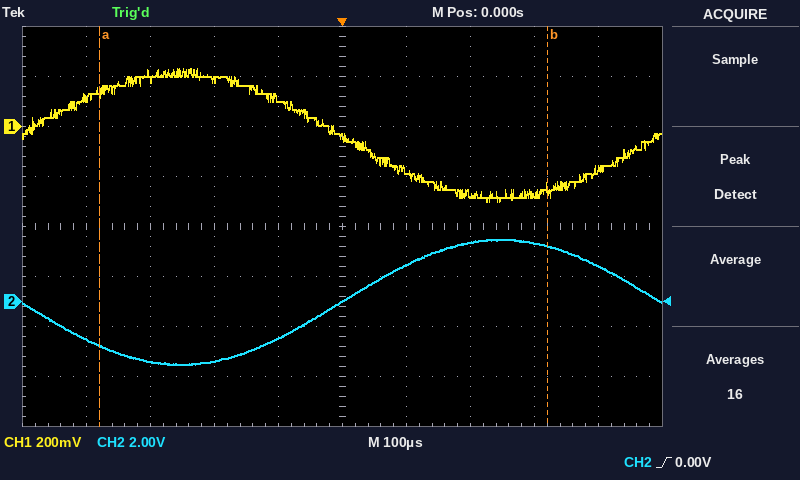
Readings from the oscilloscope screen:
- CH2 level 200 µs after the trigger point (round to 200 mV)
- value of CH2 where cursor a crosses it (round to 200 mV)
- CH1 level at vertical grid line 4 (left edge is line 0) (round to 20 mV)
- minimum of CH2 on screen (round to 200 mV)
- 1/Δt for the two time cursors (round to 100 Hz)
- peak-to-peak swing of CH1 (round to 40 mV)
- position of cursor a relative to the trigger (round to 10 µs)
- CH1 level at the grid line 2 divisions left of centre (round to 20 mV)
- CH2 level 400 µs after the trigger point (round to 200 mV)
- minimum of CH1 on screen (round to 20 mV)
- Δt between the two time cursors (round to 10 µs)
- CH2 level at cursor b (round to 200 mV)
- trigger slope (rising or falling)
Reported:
2.4 V
-1.8 V
120 mV
-2.6 V
1.4 kHz
520 mV
-380 µs
180 mV
1.4 V
-300 mV
700 µs
2.2 V
rising
